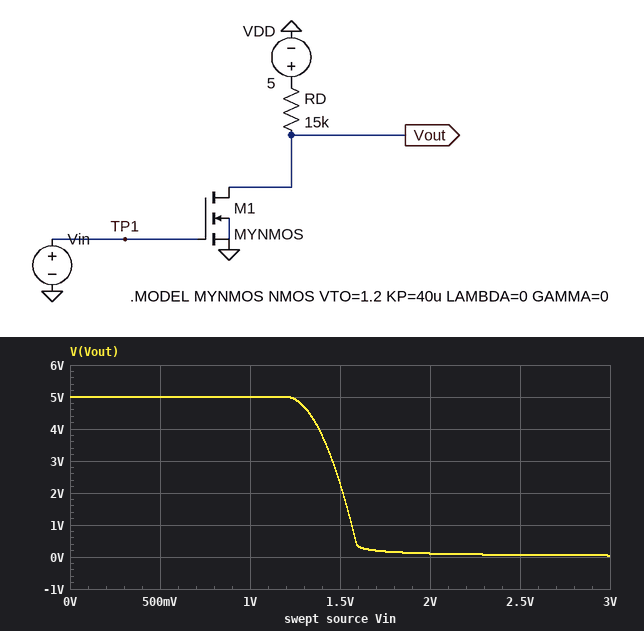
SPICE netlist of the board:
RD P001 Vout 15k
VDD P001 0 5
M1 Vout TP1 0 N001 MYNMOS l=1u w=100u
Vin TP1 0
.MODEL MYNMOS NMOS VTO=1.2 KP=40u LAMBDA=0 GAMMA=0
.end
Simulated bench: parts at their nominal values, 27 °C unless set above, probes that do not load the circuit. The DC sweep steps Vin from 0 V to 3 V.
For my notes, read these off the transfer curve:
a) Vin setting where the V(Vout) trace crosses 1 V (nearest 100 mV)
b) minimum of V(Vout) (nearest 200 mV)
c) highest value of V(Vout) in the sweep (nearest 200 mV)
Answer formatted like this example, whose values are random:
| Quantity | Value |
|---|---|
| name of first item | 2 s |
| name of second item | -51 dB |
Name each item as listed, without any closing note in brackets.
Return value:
| Quantity | Value |
|---|---|
| Vin setting where the V(Vout) trace crosses 1 V | 1.6 V |
| minimum of V(Vout) | 0 V |
| highest value of V(Vout) in the sweep | 5.0 V |
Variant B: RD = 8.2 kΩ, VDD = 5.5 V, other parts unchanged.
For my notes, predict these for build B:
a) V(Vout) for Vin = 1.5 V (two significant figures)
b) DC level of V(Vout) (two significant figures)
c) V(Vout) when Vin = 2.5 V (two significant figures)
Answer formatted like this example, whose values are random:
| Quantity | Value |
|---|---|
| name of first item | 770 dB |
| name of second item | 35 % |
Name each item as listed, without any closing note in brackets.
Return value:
| Quantity | Value |
|---|---|
| V(Vout) for Vin = 1.5 V | 4.0 V |
| DC level of V(Vout) | 5.5 V |
| V(Vout) when Vin = 2.5 V | 130 mV |
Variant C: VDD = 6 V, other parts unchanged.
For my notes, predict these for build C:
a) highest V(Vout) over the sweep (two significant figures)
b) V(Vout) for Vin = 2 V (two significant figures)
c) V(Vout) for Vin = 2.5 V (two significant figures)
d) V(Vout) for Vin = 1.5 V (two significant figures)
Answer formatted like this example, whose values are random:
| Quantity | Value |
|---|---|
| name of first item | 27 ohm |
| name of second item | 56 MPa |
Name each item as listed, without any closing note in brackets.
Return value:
| Quantity | Value |
|---|---|
| highest V(Vout) over the sweep | 6.0 V |
| V(Vout) for Vin = 2 V | 130 mV |
| V(Vout) for Vin = 2.5 V | 78 mV |
| V(Vout) for Vin = 1.5 V | 3.3 V |
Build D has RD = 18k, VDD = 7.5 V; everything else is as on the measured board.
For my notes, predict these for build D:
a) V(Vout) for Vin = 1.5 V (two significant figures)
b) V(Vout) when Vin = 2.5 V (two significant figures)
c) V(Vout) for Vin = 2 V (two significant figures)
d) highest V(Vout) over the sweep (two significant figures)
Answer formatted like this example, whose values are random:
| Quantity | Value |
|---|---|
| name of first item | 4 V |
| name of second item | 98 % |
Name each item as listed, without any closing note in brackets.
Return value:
| Quantity | Value |
|---|---|
| V(Vout) for Vin = 1.5 V | 4.3 V |
| V(Vout) when Vin = 2.5 V | 82 mV |
| V(Vout) for Vin = 2 V | 140 mV |
| highest V(Vout) over the sweep | 7.5 V |
